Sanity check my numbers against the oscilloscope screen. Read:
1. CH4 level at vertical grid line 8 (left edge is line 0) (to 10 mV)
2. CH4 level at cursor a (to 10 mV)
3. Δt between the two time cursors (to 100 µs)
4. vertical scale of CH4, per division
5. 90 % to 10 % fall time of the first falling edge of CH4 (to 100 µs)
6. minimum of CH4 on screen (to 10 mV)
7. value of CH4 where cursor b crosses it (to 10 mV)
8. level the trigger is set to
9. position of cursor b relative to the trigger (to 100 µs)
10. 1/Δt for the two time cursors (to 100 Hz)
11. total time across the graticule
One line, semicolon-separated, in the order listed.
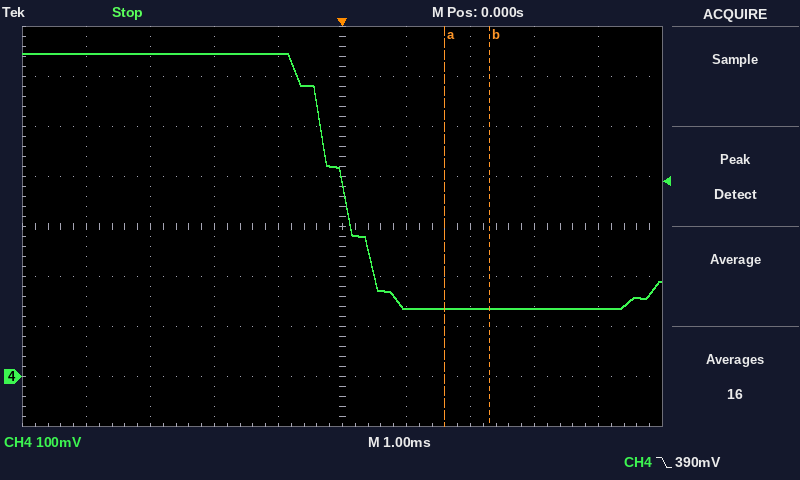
140 mV; 140 mV; 700 µs; 100 mV; 1.2 ms; 140 mV; 140 mV; 390 mV; +2.3 ms; 1.4 kHz; 10 ms
